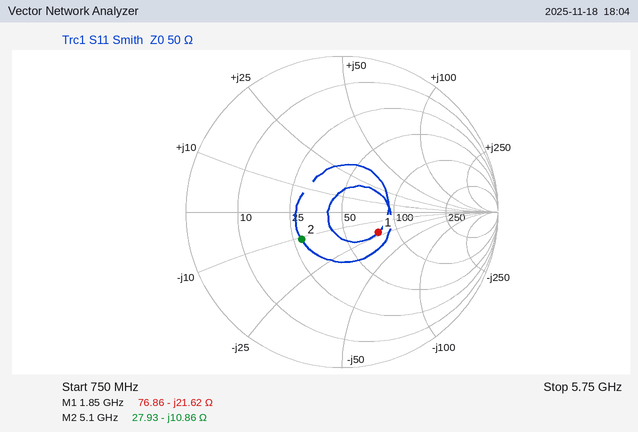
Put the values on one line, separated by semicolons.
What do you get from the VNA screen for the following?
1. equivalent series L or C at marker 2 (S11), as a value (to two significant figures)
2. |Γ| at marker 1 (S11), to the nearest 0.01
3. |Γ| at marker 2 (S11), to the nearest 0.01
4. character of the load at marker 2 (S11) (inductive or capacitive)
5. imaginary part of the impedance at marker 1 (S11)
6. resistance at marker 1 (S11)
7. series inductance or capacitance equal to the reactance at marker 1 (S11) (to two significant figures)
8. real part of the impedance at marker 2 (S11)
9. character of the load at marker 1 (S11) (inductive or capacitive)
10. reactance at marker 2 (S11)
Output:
2.9 pF; 0.27; 0.31; capacitive; -21.62 Ω; 76.86 Ω; 4.0 pF; 27.93 Ω; capacitive; -10.86 Ω
